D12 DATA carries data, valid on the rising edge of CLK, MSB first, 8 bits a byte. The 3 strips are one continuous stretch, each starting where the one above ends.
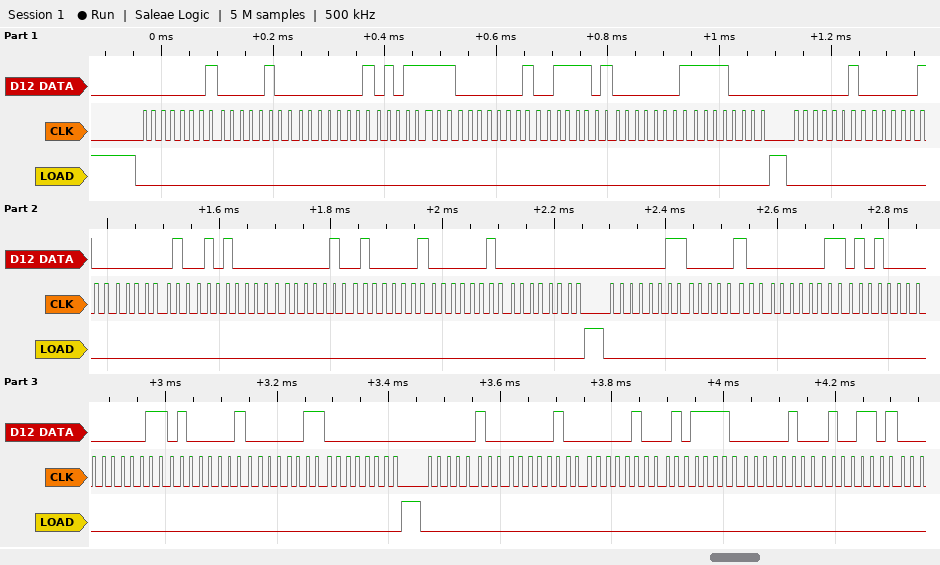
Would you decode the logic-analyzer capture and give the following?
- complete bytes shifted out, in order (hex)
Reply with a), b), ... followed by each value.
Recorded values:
a) 01 04 01 5F 01 3D 01 F0 02 04 02 50 02 41 02 00 03 04 03 50 03 41 03 00 04 04 04 5E 04 4D
